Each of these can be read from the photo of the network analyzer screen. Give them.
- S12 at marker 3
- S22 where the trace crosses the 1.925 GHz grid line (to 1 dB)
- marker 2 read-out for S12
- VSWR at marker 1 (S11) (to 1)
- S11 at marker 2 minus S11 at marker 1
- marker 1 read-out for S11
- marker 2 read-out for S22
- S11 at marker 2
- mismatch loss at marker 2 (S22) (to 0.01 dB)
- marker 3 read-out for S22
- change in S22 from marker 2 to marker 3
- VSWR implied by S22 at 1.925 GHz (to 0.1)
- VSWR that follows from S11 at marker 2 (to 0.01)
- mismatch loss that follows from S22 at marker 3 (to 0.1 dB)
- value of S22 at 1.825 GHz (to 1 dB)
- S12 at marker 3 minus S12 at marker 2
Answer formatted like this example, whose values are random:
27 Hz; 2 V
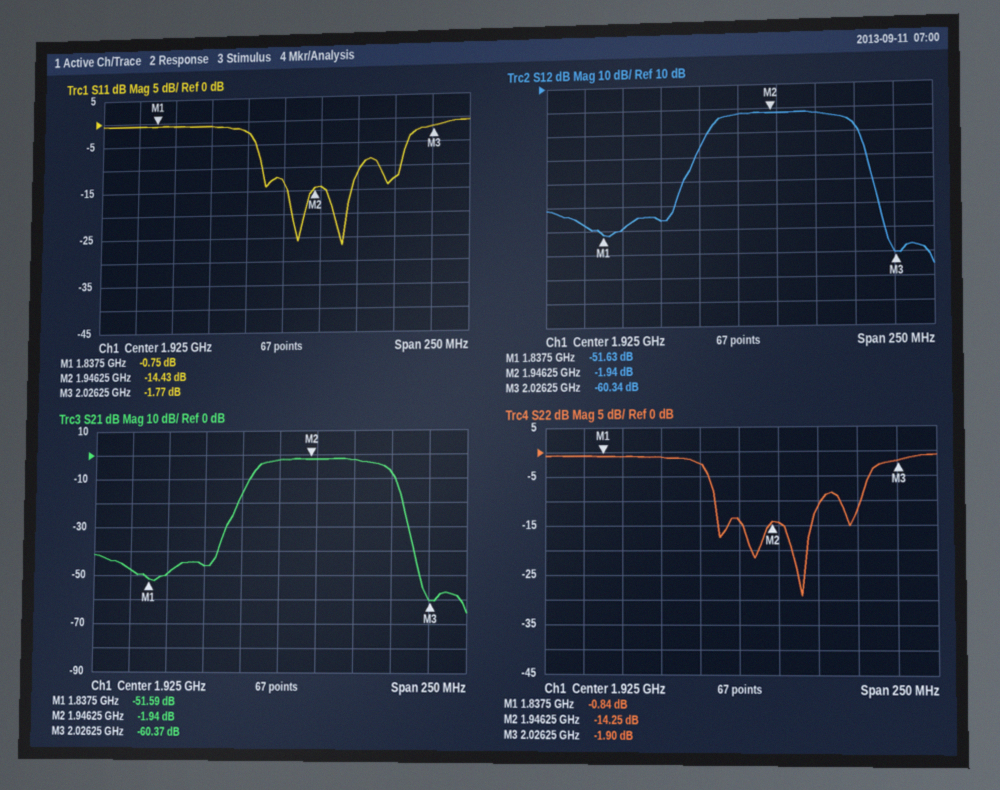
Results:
-60.34 dB; -14 dB; -1.94 dB; 23; -13.68 dB; -0.75 dB; -14.25 dB; -14.43 dB; 0.17 dB; -1.90 dB; 12.35 dB; 1.5; 1.47; 4.5 dB; -1 dB; -58.40 dB
